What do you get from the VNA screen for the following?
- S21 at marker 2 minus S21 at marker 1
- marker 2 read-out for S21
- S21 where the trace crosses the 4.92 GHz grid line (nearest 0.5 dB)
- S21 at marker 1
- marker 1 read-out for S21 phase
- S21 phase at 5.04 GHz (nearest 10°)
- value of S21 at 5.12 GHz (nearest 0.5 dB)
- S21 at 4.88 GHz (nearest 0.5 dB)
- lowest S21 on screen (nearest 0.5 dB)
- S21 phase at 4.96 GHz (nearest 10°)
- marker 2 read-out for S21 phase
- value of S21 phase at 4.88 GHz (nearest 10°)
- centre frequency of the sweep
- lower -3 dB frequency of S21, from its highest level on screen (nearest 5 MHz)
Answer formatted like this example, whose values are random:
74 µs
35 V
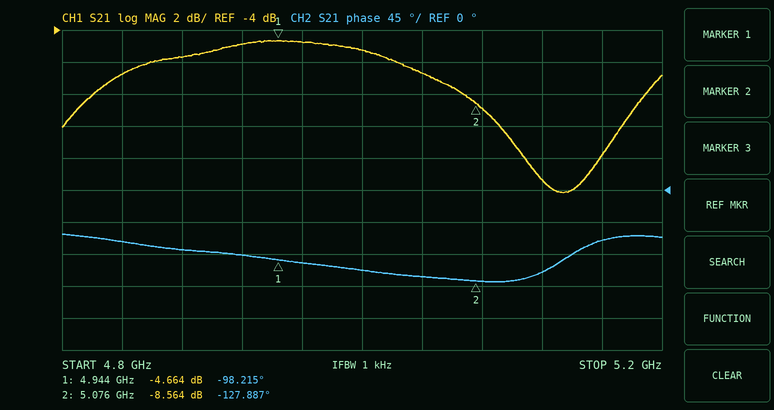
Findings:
-3.900 dB
-8.564 dB
-5.0 dB
-4.664 dB
-98.215°
-120°
-13.5 dB
-5.5 dB
-14.0 dB
-100°
-127.887°
-80°
5 GHz
4.825 GHz
